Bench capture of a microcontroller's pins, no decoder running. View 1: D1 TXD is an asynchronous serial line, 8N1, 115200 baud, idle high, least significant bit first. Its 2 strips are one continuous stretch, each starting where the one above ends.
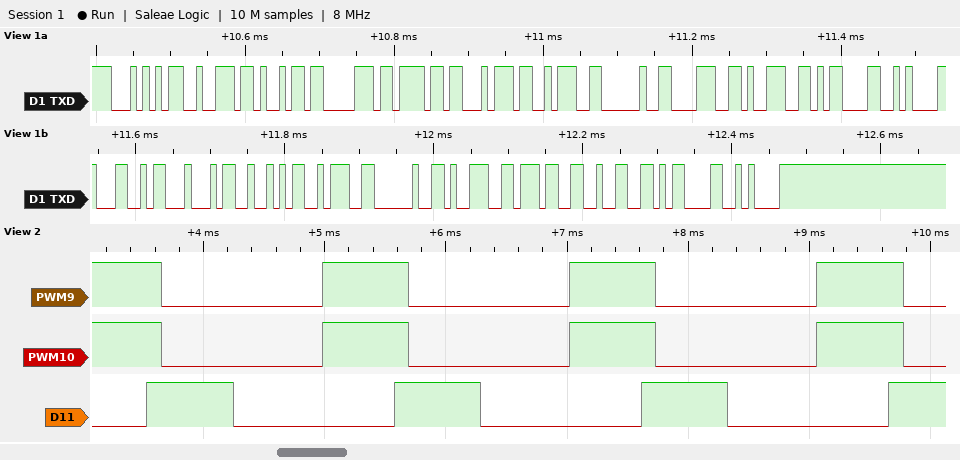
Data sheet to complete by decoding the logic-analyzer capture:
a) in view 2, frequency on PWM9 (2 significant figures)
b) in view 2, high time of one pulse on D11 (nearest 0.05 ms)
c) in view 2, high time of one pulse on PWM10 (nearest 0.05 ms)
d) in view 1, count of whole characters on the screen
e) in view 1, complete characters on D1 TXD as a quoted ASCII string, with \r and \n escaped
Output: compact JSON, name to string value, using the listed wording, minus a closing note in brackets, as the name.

{"in view 2, frequency on PWM9": "490 Hz", "in view 2, high time of one pulse on D11": "0.70 ms", "in view 2, high time of one pulse on PWM10": "0.70 ms", "in view 1, count of whole characters on the screen": "22", "in view 1, complete characters on D1 TXD as a quoted ASCII string, with \\r and \\n escaped": "\"Tripot: 89\\r\\nLDR: 972\\r\\n\""}
